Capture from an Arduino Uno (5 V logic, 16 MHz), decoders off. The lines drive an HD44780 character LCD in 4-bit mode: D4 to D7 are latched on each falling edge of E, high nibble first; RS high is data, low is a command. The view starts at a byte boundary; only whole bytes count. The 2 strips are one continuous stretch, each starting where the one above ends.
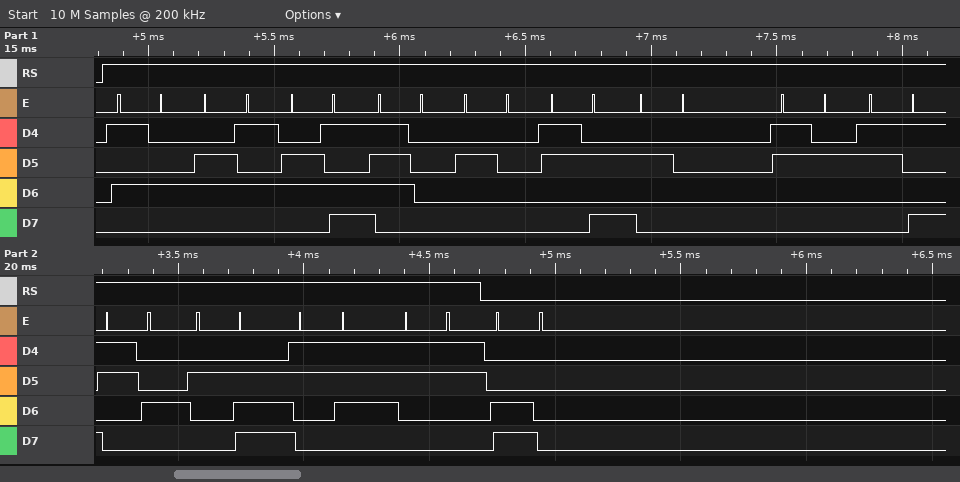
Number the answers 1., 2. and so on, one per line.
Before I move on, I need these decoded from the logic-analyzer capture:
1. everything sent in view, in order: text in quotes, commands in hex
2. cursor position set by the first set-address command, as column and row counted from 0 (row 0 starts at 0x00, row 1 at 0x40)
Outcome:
1. "Temp : 294.73" 0xC0
2. column 0, row 1
